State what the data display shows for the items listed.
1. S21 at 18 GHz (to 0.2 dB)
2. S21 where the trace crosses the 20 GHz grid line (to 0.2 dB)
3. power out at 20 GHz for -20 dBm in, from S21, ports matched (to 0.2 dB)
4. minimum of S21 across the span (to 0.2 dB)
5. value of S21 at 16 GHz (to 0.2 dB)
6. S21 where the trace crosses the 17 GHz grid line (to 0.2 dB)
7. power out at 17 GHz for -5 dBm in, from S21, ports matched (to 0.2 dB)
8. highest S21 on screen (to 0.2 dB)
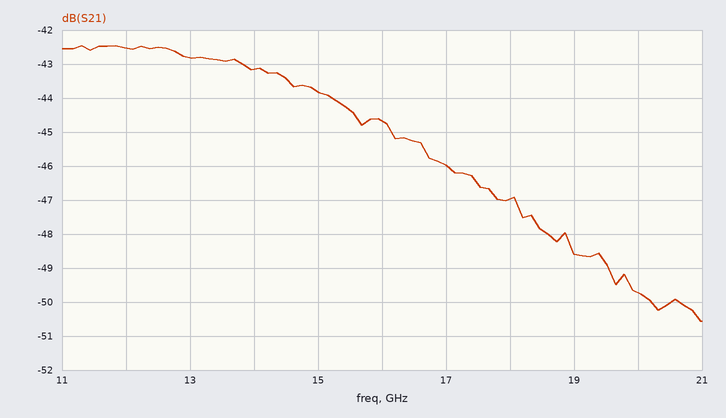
-47.0 dB
-49.8 dB
-69.8 dBm
-50.6 dB
-44.6 dB
-46.0 dB
-51.0 dBm
-42.4 dB
